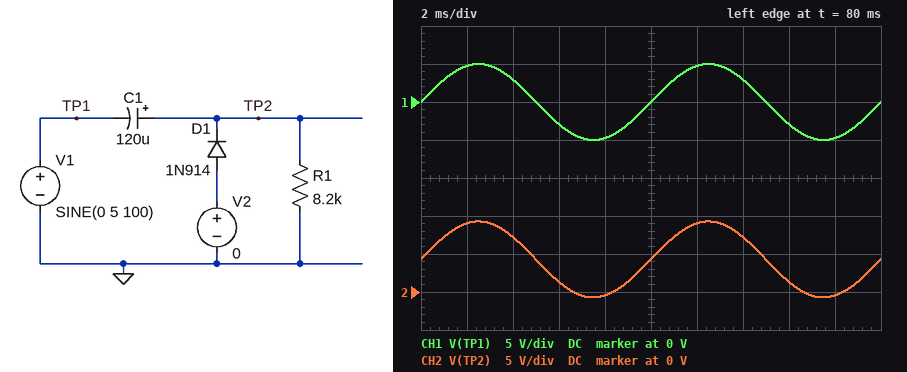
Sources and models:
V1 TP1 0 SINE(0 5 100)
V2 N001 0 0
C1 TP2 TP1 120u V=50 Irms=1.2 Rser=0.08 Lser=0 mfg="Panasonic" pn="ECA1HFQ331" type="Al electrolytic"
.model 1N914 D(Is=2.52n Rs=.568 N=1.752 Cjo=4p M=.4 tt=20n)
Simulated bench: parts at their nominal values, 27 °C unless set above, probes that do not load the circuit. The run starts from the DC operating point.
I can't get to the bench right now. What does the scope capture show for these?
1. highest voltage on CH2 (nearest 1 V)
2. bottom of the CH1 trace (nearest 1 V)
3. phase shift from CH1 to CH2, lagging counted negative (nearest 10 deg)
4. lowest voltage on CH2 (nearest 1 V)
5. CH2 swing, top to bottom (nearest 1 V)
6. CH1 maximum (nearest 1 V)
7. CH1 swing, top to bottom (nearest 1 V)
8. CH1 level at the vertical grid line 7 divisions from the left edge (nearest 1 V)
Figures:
9 V
-5 V
0 deg
-1 V
10 V
5 V
10 V
3 V
